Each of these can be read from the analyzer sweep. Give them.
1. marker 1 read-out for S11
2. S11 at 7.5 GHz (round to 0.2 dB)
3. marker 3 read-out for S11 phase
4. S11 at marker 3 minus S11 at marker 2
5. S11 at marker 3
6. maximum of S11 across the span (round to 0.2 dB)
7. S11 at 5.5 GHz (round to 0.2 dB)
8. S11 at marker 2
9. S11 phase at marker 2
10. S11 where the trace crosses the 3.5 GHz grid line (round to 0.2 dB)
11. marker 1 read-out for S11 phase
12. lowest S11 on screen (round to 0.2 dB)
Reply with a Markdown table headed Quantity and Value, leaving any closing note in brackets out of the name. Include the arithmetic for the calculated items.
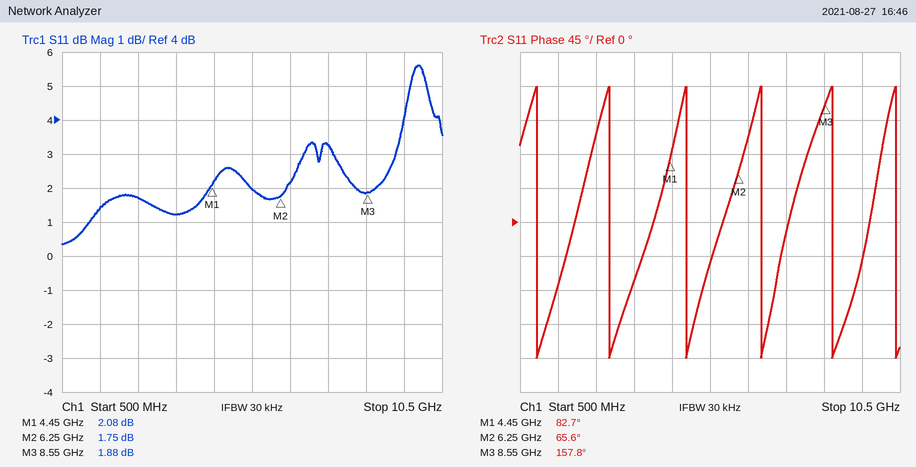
| Quantity | Value |
|---|---|
| marker 1 read-out for S11 | 2.08 dB |
| S11 at 7.5 GHz | 3.2 dB |
| marker 3 read-out for S11 phase | 157.8° |
| S11 at marker 3 minus S11 at marker 2 | 1.88 − (1.75) = 0.13 dB |
| S11 at marker 3 | 1.88 dB |
| maximum of S11 across the span | 5.6 dB |
| S11 at 5.5 GHz | 2.0 dB |
| S11 at marker 2 | 1.75 dB |
| S11 phase at marker 2 | 65.6° |
| S11 where the trace crosses the 3.5 GHz grid line | 1.2 dB |
| marker 1 read-out for S11 phase | 82.7° |
| lowest S11 on screen | 0.4 dB |
